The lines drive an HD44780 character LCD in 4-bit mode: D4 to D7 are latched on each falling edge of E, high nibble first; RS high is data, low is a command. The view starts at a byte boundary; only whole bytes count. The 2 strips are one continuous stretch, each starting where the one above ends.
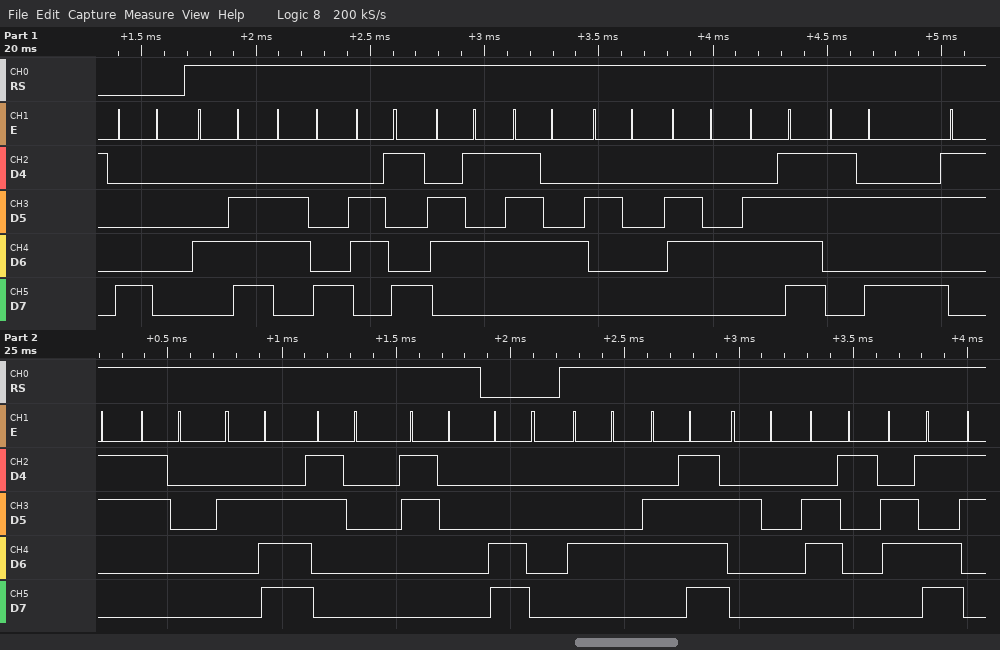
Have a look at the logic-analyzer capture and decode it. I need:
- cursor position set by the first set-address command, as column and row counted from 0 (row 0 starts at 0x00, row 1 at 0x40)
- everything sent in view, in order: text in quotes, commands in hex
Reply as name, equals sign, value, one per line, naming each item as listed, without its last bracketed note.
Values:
cursor position set by the first set-address command, as column and row counted from 0 = column 0, row 0
everything sent in view, in order: text in quotes, commands in hex = 0x80 "Nhiet do:30.00" 0xC0 "Do am"
